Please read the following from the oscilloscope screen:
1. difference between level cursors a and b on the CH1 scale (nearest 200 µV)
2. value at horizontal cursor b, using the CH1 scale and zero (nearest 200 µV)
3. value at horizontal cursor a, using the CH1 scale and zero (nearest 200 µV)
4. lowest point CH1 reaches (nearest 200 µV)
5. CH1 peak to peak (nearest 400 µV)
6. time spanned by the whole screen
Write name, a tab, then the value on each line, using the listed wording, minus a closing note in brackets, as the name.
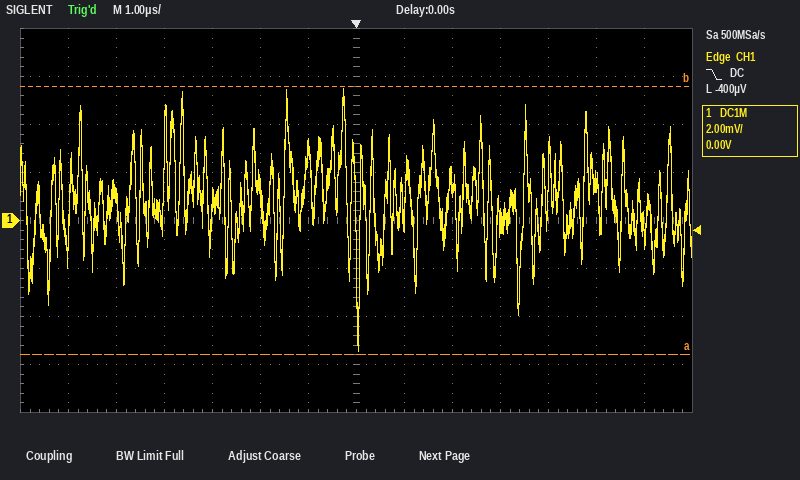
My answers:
difference between level cursors a and b on the CH1 scale	11.2 mV
value at horizontal cursor b, using the CH1 scale and zero	5.6 mV
value at horizontal cursor a, using the CH1 scale and zero	-5.6 mV
lowest point CH1 reaches	-5.4 mV
CH1 peak to peak	10.8 mV
time spanned by the whole screen	14 µs
